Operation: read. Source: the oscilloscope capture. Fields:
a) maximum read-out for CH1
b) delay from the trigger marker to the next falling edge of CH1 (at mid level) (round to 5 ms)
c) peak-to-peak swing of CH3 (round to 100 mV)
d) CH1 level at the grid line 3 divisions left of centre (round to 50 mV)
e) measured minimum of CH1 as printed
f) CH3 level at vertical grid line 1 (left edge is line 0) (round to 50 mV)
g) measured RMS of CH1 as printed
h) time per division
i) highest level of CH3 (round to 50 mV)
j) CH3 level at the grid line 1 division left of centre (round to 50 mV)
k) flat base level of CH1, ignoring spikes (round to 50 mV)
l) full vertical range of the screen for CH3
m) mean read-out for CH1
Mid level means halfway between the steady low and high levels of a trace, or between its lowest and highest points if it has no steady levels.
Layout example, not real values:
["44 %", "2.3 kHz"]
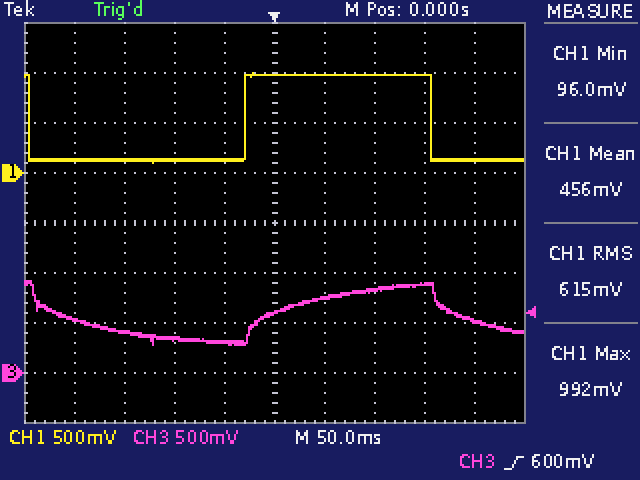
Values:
["992 mV", "155 ms", "600 mV", "150 mV", "96.0 mV", "550 mV", "615 mV", "50 ms", "900 mV", "300 mV", "150 mV", "4 V", "456 mV"]
